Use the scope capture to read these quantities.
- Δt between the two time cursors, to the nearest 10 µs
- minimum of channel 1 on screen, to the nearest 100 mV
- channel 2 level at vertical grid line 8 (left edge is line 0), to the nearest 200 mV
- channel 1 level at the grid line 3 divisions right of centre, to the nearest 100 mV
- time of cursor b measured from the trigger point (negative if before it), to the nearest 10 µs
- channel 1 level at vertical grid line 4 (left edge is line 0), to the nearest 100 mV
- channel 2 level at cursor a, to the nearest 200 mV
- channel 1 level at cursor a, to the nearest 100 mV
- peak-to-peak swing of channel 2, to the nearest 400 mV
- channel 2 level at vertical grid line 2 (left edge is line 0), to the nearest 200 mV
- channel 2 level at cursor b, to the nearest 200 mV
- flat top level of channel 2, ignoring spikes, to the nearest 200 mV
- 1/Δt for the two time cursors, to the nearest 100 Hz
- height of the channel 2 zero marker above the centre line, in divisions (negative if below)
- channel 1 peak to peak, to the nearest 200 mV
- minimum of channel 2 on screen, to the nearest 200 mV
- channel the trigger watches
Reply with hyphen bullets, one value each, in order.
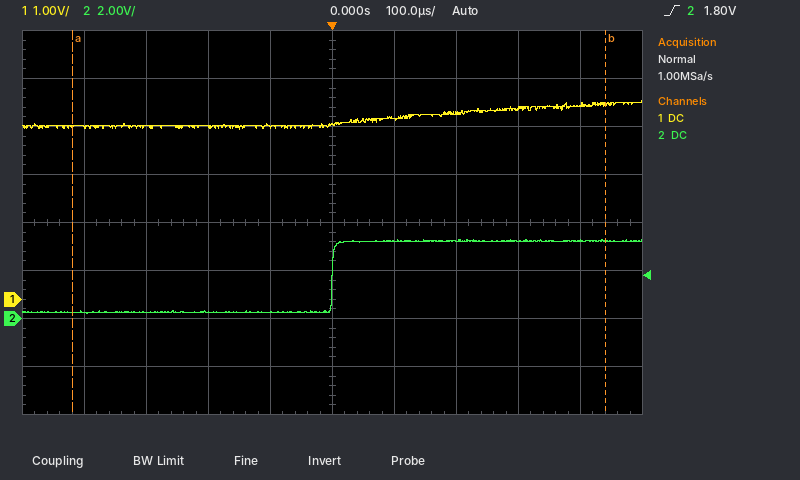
- 860 µs
- 3.5 V
- 3.2 V
- 4.0 V
- +440 µs
- 3.6 V
- 200 mV
- 3.6 V
- 3.2 V
- 200 mV
- 3.2 V
- 3.2 V
- 1.2 kHz
- -2.0 div
- 600 mV
- 200 mV
- channel 2
